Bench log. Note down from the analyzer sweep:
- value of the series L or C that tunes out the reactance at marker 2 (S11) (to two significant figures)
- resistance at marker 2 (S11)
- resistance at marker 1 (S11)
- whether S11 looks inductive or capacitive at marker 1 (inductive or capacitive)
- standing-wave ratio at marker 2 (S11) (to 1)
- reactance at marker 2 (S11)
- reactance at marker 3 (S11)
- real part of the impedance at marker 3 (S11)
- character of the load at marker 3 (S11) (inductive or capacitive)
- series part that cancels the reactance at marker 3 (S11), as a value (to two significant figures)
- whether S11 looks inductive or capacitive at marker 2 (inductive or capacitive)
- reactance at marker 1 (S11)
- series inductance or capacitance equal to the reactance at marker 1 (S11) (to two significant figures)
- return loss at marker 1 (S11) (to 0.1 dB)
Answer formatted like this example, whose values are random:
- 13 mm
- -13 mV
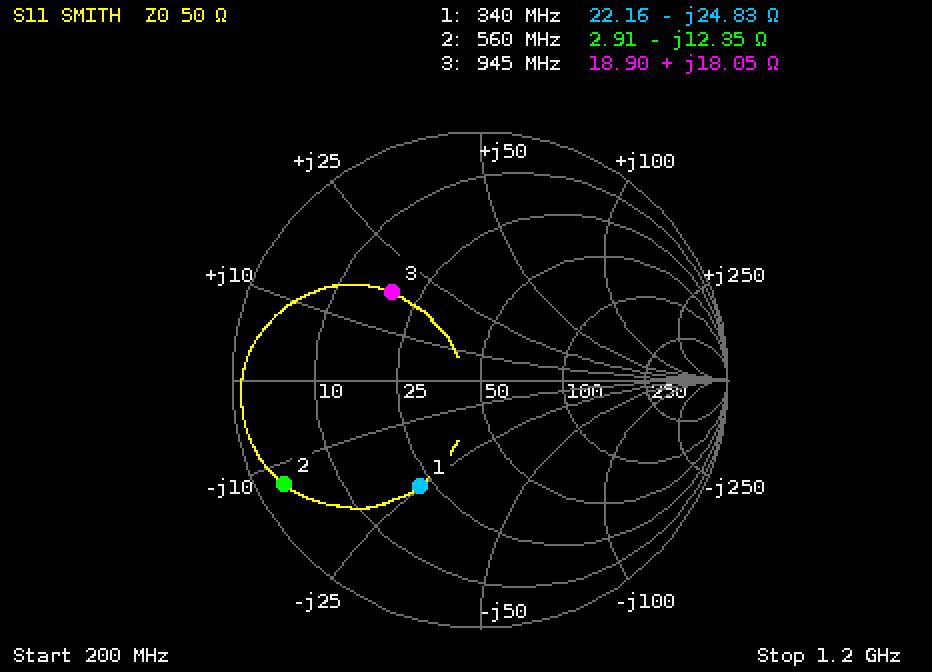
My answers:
- 3.5 nH
- 2.91 Ω
- 22.16 Ω
- capacitive
- 18
- -12.35 Ω
- +18.05 Ω
- 18.90 Ω
- inductive
- 9.3 pF
- capacitive
- -24.83 Ω
- 19 pF
- 6.2 dB
